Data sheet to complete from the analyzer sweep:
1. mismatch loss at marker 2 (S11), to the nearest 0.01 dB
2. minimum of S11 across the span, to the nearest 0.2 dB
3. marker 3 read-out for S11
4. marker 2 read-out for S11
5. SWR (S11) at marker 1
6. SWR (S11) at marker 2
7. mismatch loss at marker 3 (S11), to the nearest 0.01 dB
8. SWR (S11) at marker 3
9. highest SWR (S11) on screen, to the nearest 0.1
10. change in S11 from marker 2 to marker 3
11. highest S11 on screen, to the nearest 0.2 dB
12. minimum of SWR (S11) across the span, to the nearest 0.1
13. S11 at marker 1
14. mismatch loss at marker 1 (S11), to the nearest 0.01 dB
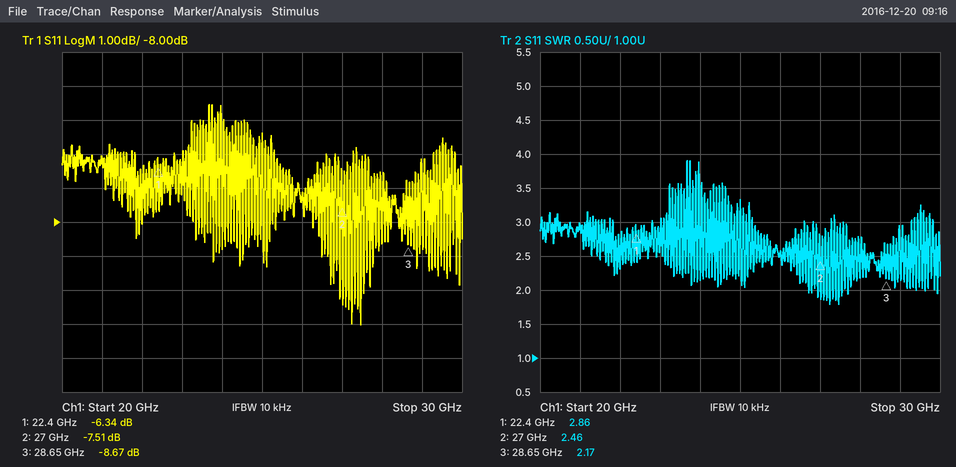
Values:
0.85 dB
-11.0 dB
-8.67 dB
-7.51 dB
2.86
2.46
0.63 dB
2.17
3.9
-1.16 dB
-4.6 dB
1.8
-6.34 dB
1.15 dB
